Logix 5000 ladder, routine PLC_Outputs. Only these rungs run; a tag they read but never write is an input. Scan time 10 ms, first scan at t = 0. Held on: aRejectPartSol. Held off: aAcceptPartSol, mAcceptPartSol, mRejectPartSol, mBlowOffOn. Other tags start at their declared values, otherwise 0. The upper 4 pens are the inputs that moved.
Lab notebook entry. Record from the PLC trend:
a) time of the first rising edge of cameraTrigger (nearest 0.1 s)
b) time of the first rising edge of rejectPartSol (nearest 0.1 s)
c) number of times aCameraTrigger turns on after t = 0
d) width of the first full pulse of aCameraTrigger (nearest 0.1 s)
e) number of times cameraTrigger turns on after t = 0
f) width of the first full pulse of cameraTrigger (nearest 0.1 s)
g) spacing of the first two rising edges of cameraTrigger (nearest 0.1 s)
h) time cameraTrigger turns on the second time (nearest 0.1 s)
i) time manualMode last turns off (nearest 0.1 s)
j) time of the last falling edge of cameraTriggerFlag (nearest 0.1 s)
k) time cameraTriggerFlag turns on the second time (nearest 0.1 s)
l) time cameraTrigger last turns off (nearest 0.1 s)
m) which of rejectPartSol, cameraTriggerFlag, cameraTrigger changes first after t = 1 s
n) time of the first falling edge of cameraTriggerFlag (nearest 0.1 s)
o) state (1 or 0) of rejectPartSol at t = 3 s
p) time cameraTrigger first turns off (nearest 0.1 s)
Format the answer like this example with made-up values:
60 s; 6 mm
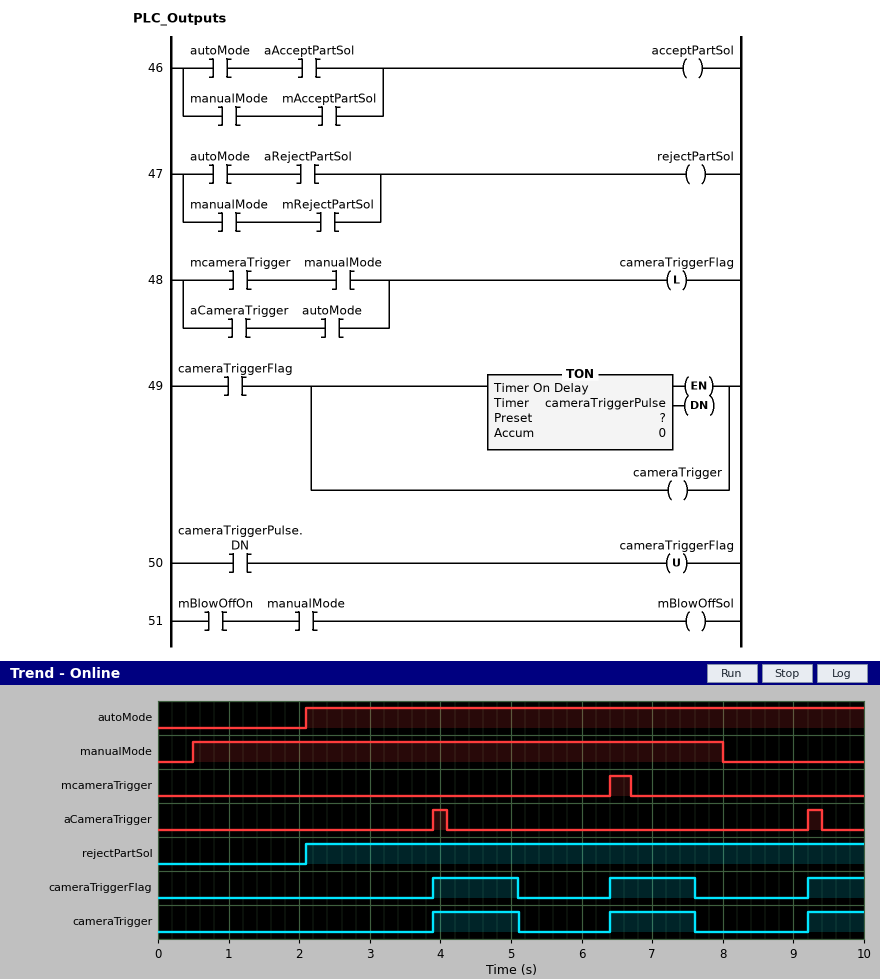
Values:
3.9 s; 2.1 s; 2; 0.2 s; 3; 1.2 s; 2.5 s; 6.4 s; 8.0 s; 7.6 s; 6.4 s; 7.6 s; rejectPartSol; 5.1 s; 1; 5.1 s
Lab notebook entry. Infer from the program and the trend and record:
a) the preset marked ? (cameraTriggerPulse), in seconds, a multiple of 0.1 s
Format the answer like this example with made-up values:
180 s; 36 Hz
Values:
1.2 s
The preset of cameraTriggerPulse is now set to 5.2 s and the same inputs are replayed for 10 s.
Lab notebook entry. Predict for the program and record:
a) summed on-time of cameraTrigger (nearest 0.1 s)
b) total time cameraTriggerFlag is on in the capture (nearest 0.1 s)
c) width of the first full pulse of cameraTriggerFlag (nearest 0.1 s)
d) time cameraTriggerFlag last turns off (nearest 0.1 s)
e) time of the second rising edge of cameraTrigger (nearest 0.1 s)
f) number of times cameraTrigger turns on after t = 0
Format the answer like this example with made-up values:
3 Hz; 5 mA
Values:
6.0 s; 6.0 s; 5.2 s; 9.1 s; 9.2 s; 2
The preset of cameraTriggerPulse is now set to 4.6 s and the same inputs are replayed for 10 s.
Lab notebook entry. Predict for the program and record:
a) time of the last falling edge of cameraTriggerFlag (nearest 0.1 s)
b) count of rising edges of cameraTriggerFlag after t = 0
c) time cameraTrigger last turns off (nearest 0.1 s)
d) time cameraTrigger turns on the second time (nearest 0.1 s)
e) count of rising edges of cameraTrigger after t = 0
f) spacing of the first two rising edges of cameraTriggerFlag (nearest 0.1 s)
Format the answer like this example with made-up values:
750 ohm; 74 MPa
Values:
8.5 s; 2; 8.5 s; 9.2 s; 2; 5.3 s
